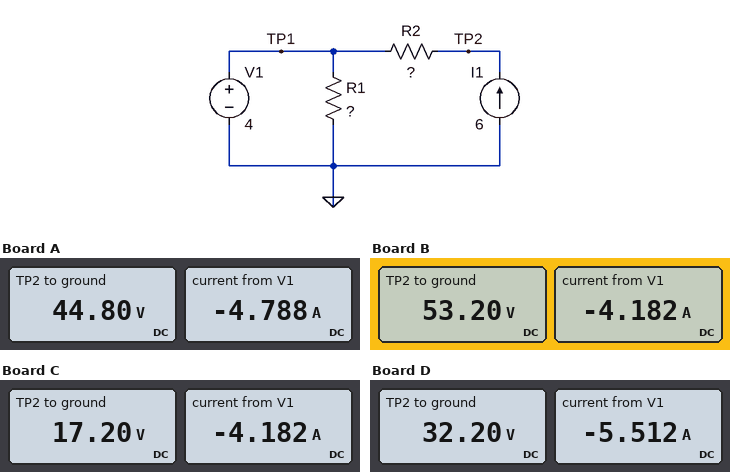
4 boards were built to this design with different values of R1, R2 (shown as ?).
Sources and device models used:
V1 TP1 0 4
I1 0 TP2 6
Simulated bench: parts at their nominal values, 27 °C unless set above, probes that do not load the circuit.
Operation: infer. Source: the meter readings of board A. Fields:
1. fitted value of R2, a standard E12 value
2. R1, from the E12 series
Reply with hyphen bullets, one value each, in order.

- 6.8 Ω
- 3.3 Ω
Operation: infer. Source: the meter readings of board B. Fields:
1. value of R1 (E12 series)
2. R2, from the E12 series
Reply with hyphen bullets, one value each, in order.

- 2.2 Ω
- 8.2 Ω
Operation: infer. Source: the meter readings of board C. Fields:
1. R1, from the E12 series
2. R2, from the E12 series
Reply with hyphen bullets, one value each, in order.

- 2.2 Ω
- 2.2 Ω
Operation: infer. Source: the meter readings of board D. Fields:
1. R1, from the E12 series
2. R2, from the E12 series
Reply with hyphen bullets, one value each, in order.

- 8.2 Ω
- 4.7 Ω
